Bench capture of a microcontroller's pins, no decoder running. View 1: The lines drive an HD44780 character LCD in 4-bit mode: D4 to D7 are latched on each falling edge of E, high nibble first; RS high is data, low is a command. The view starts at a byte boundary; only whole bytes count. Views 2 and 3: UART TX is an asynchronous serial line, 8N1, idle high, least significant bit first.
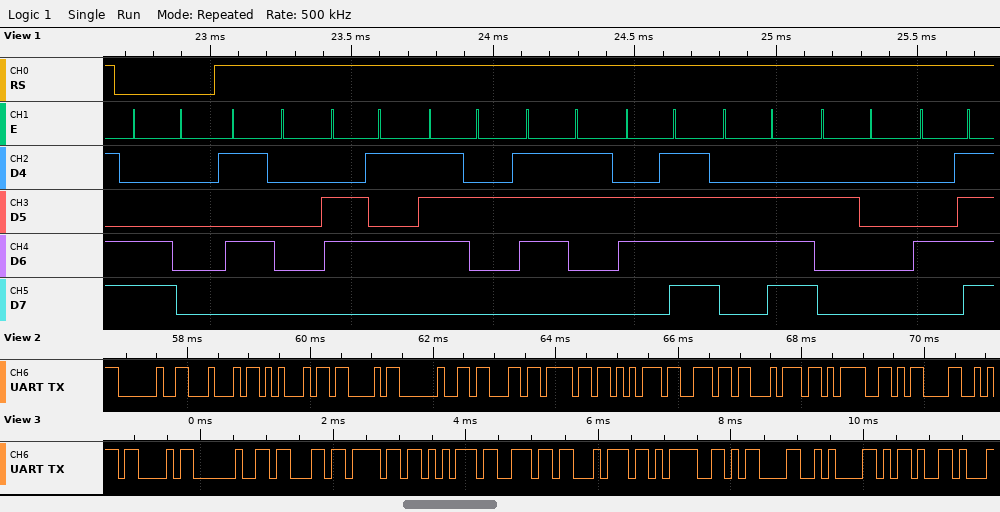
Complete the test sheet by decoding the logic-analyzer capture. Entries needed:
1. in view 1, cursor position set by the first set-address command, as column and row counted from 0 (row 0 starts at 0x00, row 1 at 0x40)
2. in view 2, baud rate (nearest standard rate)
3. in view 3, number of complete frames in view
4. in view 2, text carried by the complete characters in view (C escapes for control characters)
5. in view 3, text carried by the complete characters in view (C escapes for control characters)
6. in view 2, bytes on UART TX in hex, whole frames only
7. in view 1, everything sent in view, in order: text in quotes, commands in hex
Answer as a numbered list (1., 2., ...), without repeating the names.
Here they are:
1. column 0, row 1
2. 9600 baud
3. 11
4. " DEC count=\r"
5. "C count=\r\n-"
6. 20 44 45 43 20 63 6F 75 6E 74 3D 0D
7. 0xC0 "Person O"
